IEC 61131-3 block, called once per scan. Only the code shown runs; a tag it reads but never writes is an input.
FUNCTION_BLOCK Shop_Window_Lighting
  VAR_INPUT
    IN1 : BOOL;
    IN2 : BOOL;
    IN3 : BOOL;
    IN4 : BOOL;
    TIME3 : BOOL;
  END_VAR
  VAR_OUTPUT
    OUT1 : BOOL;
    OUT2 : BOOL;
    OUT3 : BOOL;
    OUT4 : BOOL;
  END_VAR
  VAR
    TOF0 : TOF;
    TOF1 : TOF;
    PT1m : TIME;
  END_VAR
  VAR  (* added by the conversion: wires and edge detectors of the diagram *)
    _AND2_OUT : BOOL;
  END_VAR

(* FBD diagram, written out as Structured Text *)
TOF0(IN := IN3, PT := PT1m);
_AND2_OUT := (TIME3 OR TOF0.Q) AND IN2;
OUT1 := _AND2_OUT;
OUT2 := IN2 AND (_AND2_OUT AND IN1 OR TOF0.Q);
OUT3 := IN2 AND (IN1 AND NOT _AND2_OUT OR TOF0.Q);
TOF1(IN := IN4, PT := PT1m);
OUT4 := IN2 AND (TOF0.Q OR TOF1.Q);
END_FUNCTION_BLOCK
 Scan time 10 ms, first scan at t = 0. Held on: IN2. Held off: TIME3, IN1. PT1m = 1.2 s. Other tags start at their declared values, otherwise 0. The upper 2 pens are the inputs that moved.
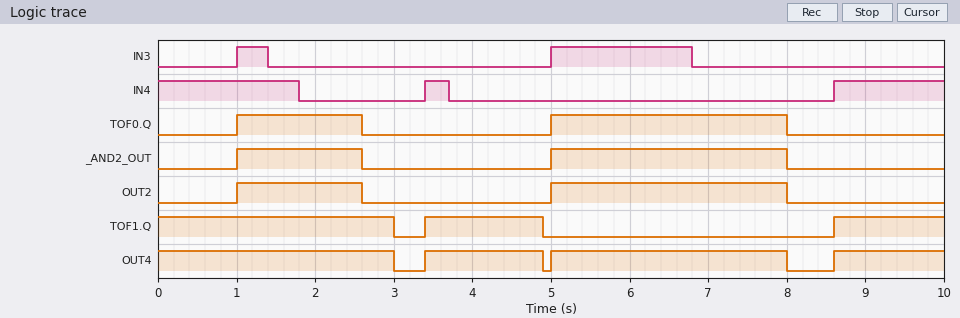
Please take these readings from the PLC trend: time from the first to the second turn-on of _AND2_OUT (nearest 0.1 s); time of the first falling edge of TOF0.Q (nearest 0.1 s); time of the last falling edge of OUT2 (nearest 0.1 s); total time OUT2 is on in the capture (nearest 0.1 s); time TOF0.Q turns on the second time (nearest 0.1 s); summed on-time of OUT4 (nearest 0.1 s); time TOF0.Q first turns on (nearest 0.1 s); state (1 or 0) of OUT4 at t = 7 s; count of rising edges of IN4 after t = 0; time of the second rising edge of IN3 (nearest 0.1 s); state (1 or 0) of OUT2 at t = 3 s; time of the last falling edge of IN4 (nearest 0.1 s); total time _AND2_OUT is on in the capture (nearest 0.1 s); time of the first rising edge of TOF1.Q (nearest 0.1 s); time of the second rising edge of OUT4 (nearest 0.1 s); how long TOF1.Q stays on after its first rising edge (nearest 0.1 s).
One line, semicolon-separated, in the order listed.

4.0 s; 2.6 s; 8.0 s; 4.6 s; 5.0 s; 8.9 s; 1.0 s; 1; 2; 5.0 s; 0; 3.7 s; 4.6 s; 3.4 s; 5.0 s; 1.5 s
